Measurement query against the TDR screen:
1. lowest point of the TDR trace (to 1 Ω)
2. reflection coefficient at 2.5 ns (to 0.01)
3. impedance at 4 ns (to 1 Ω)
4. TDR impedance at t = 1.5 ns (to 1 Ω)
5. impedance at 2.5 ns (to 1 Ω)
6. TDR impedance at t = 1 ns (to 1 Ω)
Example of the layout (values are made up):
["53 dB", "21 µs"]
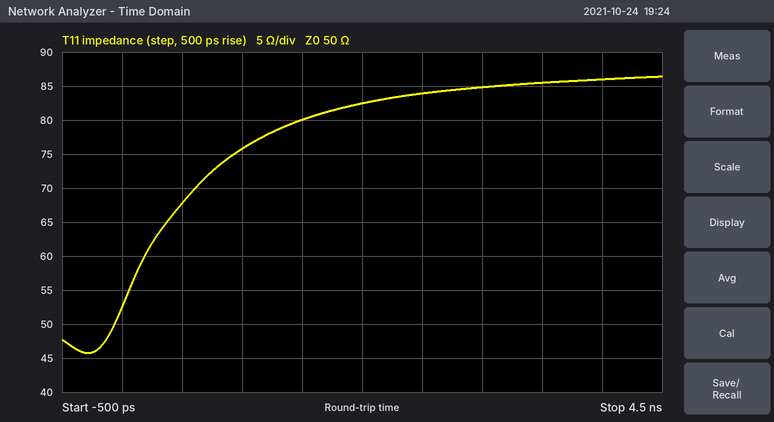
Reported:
["46 Ω", "+0.25", "86 Ω", "80 Ω", "84 Ω", "76 Ω"]
